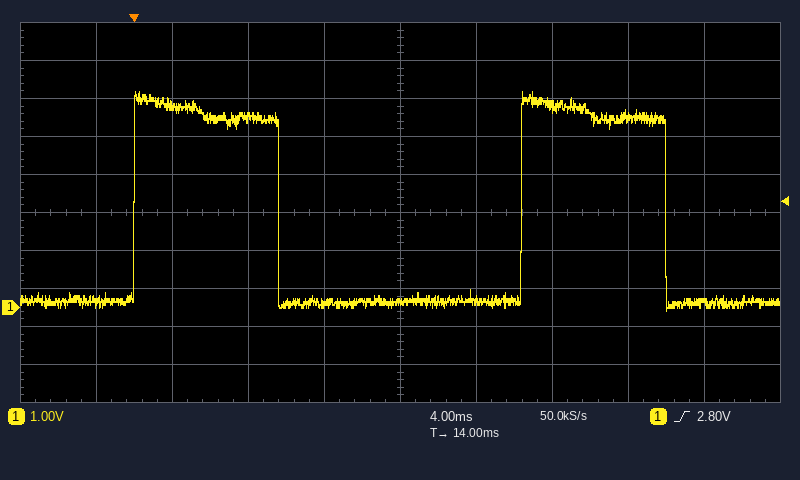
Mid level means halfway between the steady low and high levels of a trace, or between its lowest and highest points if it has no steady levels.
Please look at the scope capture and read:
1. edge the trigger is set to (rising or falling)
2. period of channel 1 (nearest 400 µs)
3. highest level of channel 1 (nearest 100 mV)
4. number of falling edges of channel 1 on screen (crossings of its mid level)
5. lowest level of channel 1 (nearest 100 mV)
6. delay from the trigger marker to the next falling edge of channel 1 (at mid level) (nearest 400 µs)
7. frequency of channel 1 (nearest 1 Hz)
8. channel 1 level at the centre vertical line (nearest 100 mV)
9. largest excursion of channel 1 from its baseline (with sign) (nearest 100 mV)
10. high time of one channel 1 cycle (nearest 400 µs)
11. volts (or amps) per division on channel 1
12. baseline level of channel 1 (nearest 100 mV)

rising
20.4 ms
5.7 V
2
-100 mV
7.6 ms
49 Hz
200 mV
+5.5 V
7.6 ms
1 V
200 mV
